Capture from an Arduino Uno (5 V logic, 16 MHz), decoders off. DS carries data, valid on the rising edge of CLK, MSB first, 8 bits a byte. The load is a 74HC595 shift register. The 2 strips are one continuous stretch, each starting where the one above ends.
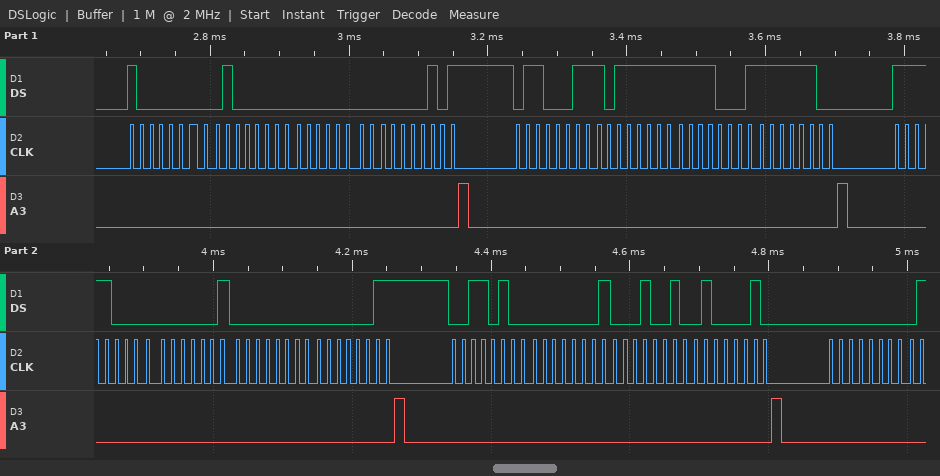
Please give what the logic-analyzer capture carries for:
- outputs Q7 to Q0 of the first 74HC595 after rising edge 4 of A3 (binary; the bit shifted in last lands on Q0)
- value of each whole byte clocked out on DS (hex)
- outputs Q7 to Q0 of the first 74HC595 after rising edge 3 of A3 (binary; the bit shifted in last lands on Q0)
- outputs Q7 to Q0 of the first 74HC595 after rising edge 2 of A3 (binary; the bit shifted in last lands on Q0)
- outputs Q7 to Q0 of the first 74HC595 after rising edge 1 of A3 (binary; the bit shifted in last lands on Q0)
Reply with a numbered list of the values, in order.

1. 01000010
2. 0x80 0x40 0x00 0x05 0x63 0xBF 0xF1 0xFC 0xF8 0x01 0x00 0x03 0x34 0x01 0x12 0x42 0x00
3. 00000011
4. 11111100
5. 00000101
